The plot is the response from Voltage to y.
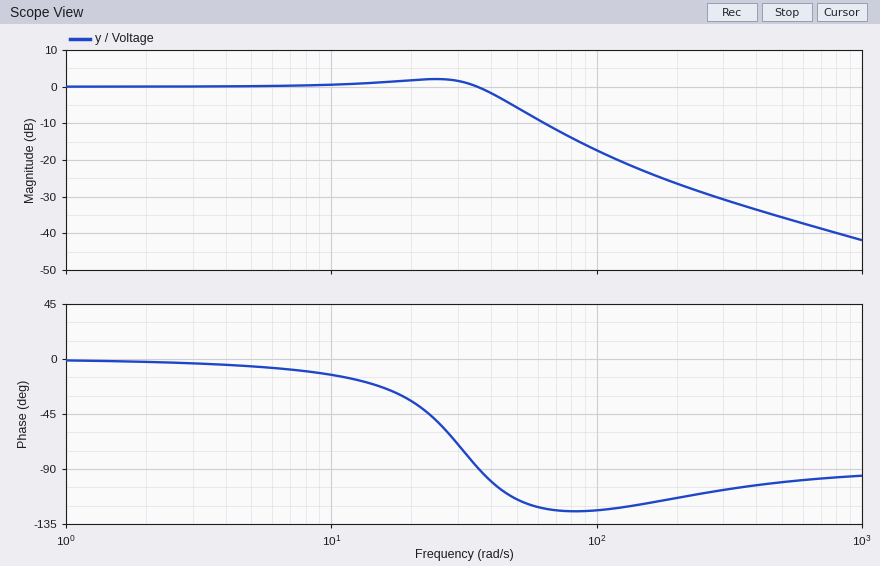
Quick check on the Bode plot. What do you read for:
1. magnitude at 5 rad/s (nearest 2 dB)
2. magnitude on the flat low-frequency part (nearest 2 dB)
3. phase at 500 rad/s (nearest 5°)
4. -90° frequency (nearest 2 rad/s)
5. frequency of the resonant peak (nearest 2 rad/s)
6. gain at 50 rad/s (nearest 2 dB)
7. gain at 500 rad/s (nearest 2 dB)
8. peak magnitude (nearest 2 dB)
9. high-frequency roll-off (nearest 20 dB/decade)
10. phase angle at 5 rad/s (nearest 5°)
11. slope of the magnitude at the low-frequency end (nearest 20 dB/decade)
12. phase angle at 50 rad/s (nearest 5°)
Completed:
0 dB
0 dB
-100°
36 rad/s
24 rad/s
-6 dB
-36 dB
2 dB
-20 dB/decade
-5°
0 dB/decade
-115°
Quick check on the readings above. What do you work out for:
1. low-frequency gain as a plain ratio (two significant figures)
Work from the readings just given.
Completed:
1.0
